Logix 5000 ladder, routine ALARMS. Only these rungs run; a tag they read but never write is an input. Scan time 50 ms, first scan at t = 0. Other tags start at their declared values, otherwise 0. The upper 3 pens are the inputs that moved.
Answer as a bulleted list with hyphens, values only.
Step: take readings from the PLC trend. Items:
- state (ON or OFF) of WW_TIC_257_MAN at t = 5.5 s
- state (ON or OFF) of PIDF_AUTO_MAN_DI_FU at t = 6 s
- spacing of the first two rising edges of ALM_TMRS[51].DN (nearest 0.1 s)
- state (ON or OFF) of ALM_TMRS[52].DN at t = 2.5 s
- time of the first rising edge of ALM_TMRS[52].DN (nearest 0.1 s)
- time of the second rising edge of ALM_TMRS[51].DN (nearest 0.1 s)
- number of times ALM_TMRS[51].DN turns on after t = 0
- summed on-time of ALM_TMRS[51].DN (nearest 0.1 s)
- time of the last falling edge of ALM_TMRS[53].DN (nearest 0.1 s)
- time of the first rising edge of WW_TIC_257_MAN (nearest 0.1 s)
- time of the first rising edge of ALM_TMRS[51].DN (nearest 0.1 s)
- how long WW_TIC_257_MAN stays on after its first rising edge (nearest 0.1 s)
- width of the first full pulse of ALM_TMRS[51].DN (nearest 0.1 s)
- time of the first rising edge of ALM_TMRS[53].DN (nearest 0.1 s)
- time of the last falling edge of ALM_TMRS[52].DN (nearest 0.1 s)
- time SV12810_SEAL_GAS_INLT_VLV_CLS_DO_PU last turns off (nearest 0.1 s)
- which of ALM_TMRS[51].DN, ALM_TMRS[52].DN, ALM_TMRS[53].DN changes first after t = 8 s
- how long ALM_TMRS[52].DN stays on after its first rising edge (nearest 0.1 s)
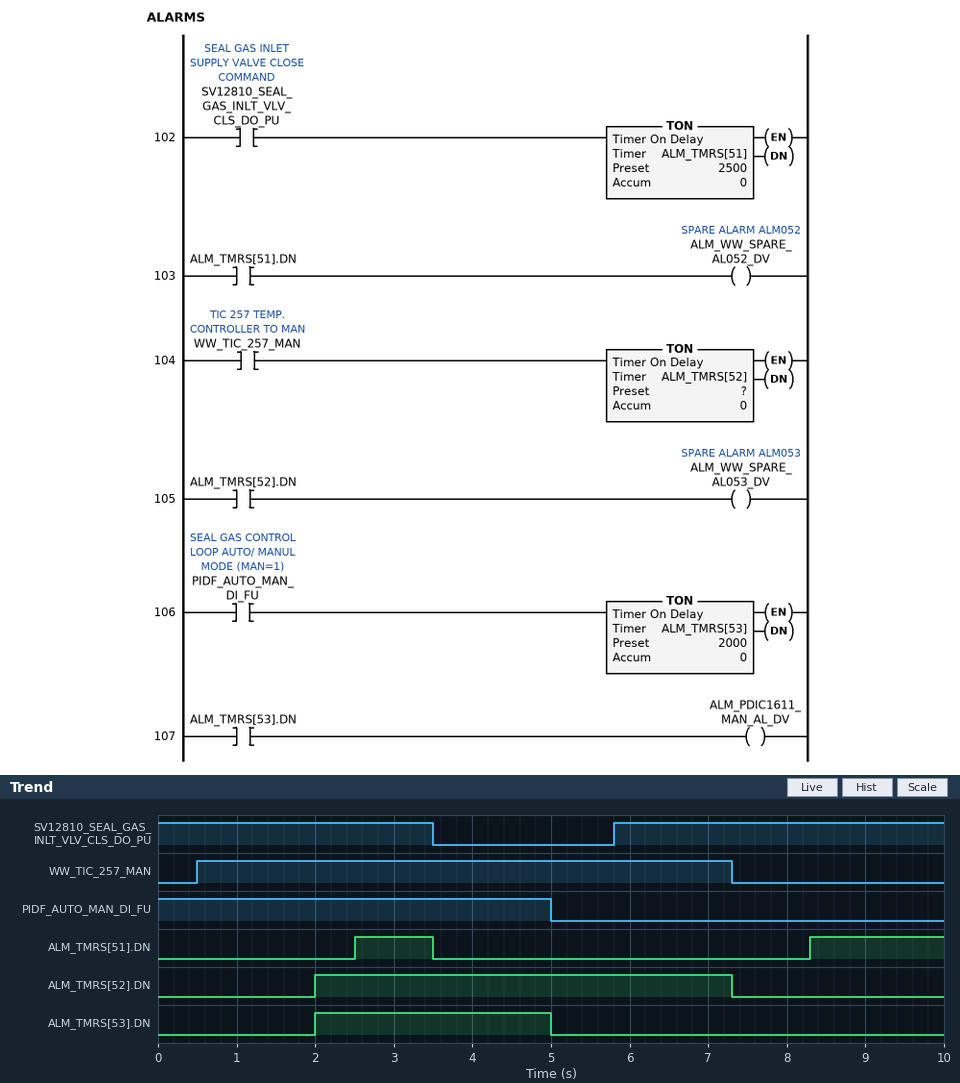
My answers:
- ON
- OFF
- 5.8 s
- ON
- 2.0 s
- 8.3 s
- 2
- 2.7 s
- 5.0 s
- 0.5 s
- 2.5 s
- 6.8 s
- 1.0 s
- 2.0 s
- 7.3 s
- 3.5 s
- ALM_TMRS[51].DN
- 5.3 s
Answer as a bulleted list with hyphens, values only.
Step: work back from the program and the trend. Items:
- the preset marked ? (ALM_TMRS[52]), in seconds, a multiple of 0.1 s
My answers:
- 1.5 s
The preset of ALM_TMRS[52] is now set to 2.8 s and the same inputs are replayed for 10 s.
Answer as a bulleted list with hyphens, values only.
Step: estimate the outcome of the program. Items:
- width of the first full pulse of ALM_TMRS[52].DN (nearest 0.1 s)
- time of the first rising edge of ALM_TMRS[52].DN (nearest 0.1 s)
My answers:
- 4.0 s
- 3.3 s
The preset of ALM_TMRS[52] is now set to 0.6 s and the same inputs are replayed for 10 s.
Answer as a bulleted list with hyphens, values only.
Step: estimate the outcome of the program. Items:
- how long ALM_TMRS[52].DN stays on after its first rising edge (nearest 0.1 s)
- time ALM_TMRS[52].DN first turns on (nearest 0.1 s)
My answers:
- 6.2 s
- 1.1 s
